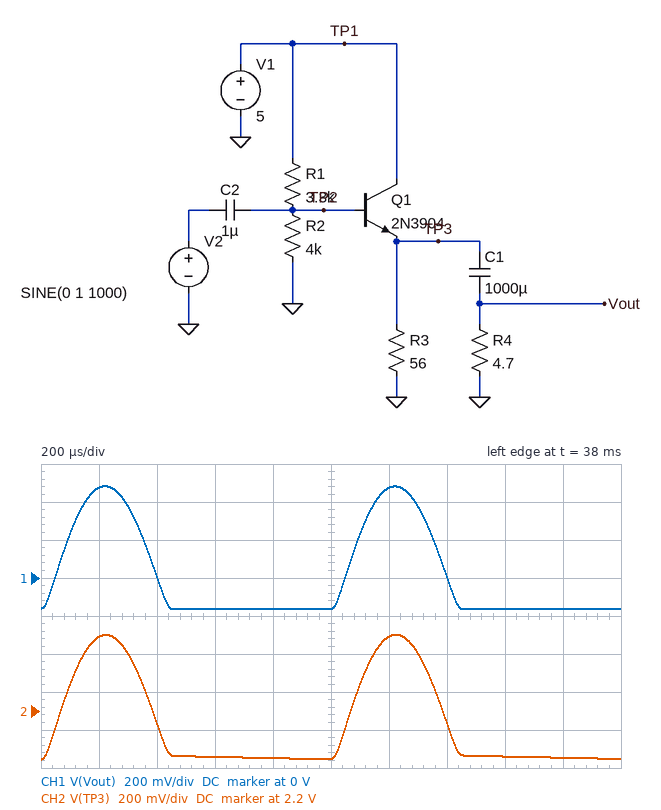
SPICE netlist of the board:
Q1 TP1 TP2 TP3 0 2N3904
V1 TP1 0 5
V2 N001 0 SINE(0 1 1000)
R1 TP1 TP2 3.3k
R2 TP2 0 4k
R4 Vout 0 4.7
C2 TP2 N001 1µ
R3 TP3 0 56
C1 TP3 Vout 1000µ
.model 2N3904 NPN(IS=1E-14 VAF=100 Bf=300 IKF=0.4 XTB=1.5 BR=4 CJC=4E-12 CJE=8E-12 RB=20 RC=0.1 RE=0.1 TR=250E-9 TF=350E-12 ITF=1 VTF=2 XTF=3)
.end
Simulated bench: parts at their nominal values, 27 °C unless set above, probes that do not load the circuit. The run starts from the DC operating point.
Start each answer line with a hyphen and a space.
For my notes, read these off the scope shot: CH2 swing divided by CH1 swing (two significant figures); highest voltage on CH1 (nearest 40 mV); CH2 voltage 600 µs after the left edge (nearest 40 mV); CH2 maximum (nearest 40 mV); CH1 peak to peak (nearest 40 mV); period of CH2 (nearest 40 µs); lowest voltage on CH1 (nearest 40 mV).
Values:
- 1.0
- 480 mV
- 1.96 V
- 2.60 V
- 640 mV
- 1.00 ms
- -160 mV
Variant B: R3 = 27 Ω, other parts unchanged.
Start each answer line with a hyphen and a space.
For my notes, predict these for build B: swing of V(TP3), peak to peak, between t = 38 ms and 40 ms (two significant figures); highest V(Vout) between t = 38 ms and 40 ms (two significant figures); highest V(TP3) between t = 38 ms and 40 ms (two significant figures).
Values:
- 850 mV
- 580 mV
- 2.3 V
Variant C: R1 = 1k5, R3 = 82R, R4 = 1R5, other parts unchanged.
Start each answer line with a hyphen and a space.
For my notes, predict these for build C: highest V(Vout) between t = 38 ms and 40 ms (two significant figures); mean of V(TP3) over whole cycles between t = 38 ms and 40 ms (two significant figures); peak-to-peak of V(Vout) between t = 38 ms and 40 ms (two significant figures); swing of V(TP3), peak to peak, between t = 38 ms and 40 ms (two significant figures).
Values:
- 250 mV
- 3.3 V
- 310 mV
- 320 mV
